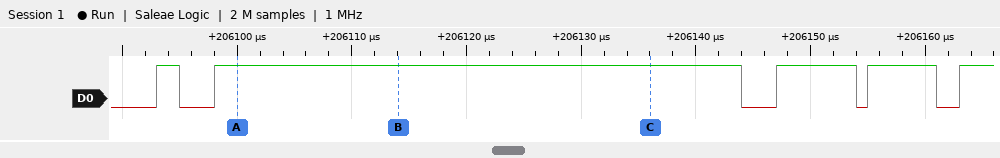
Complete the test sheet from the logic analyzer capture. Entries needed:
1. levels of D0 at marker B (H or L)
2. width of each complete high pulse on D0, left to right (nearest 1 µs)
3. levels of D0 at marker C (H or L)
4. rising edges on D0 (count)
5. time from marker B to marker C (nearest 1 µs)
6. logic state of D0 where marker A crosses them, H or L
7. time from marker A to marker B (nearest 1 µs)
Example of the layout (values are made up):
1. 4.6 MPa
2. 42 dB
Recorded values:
1. D0=H
2. 2 µs, 46 µs, 7 µs, 6 µs
3. D0=H
4. 5
5. 22 µs
6. D0=H
7. 14 µs
